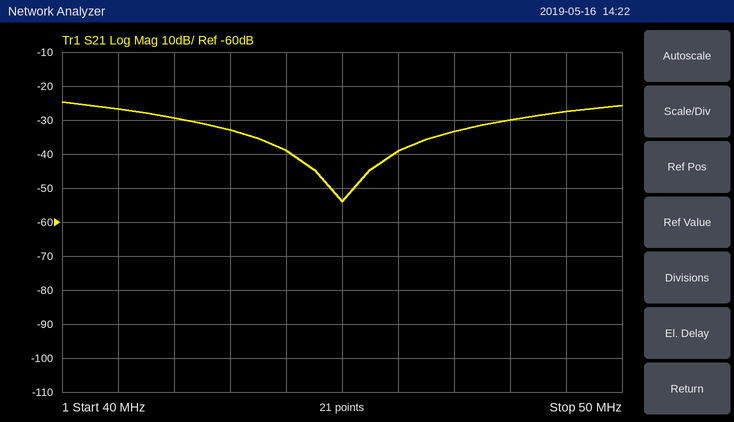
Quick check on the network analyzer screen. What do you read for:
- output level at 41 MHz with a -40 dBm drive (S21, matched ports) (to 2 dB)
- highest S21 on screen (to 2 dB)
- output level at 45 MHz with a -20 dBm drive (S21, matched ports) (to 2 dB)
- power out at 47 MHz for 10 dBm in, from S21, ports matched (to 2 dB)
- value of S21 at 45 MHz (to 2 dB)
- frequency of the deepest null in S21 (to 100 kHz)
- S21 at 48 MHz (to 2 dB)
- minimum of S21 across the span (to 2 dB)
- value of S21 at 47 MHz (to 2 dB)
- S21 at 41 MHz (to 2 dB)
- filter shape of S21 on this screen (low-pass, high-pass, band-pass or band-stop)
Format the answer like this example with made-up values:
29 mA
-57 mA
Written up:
-66 dBm
-24 dB
-74 dBm
-24 dBm
-54 dB
45.0 MHz
-30 dB
-54 dB
-34 dB
-26 dB
band-stop
